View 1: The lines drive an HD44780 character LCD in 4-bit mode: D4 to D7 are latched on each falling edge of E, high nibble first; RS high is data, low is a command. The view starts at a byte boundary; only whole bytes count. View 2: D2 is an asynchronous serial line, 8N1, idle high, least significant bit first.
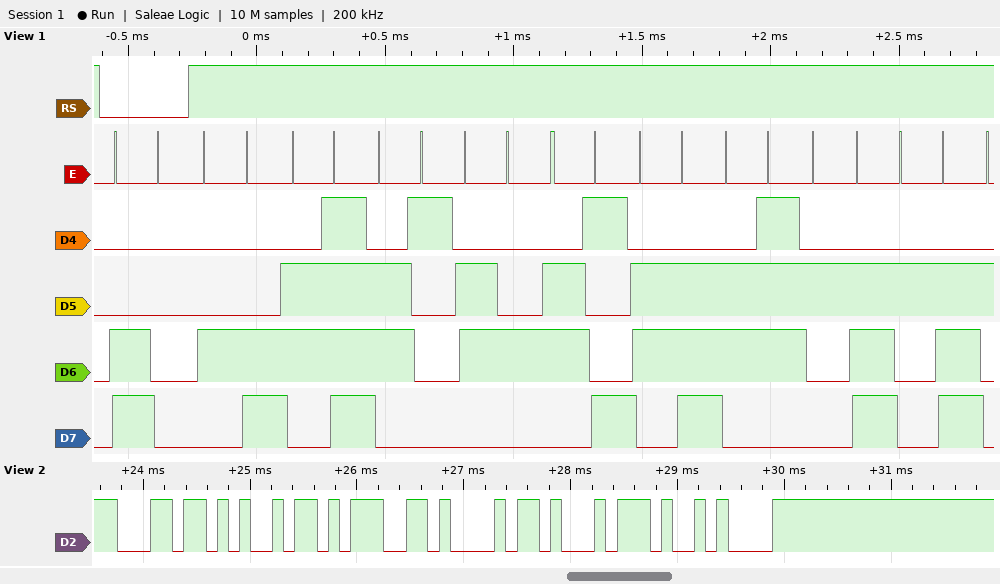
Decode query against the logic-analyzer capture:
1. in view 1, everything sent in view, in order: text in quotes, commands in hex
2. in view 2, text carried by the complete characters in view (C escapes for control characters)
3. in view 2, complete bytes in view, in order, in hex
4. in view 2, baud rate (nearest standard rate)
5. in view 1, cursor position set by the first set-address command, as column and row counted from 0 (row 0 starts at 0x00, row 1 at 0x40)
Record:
0xC0 "Loading.."
"light\n"
0x6C 0x69 0x67 0x68 0x74 0x0A
9600 baud
column 0, row 1
